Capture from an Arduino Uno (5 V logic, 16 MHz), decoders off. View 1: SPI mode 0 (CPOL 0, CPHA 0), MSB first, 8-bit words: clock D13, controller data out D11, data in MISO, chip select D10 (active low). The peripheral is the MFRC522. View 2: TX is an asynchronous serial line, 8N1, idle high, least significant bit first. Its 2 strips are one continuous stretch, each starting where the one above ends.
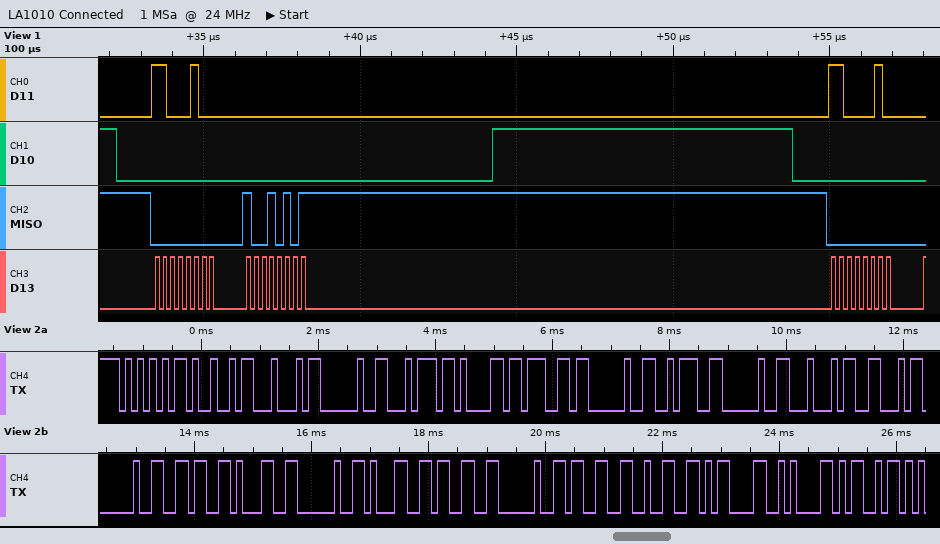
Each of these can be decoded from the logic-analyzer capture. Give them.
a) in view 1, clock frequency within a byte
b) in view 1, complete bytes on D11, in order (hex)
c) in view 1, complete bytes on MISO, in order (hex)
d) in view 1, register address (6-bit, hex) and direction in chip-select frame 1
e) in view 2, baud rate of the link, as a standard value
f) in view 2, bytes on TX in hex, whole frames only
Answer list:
4 MHz
C4 00 C2
00 95 00
0x22 read
9600 baud
55 49 44 20 74 61 67 20 3A 20 44 46 20 36 31 20 31 33 20 33 32 0D 0A 4D
